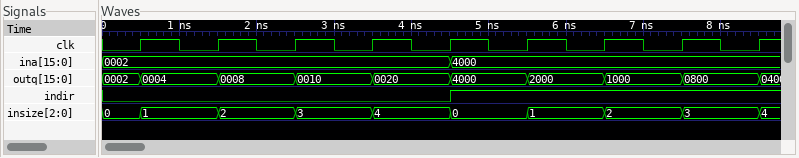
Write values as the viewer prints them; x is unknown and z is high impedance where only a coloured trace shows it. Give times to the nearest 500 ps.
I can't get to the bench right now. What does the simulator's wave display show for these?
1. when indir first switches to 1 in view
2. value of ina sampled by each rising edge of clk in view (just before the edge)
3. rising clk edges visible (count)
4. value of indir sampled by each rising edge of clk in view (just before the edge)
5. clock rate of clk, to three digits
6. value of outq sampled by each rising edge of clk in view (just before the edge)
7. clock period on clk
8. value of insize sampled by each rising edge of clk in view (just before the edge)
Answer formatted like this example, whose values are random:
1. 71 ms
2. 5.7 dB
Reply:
1. 4500 ps
2. 0002, 0002, 0002, 0002, 0002, 4000, 4000, 4000, 4000
3. 9
4. 0 0 0 0 0 1 1 1 1
5. 1.00 GHz
6. 0002, 0004, 0008, 0010, 0020, 4000, 2000, 1000, 0800
7. 1000 ps
8. 0, 1, 2, 3, 4, 0, 1, 2, 3
